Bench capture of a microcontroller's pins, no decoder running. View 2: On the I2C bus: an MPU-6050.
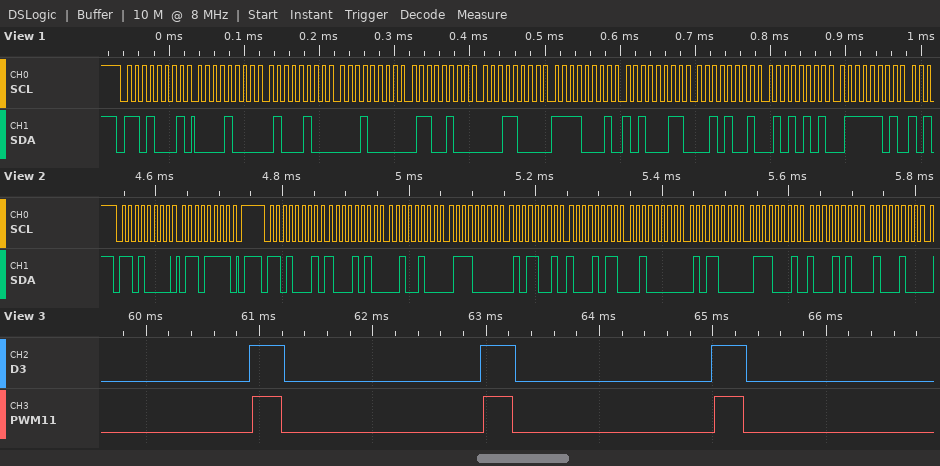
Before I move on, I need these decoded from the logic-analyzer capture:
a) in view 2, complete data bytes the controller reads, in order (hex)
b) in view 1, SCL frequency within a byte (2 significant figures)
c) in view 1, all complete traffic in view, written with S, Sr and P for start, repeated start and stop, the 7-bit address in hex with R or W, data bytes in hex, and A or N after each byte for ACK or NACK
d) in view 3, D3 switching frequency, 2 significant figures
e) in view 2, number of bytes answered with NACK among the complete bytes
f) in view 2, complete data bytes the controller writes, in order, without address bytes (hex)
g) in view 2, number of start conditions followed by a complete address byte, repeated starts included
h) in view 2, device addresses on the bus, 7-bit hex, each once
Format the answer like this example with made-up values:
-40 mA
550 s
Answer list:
8A 24 70 59 8B 20 58 71 8A 44
100 kHz
S 68R A 08 A 44 A 10 A 64 A 18 A F1 A A3 A 29 A 55 A 7D A
490 Hz
0
6F
2
0x68
